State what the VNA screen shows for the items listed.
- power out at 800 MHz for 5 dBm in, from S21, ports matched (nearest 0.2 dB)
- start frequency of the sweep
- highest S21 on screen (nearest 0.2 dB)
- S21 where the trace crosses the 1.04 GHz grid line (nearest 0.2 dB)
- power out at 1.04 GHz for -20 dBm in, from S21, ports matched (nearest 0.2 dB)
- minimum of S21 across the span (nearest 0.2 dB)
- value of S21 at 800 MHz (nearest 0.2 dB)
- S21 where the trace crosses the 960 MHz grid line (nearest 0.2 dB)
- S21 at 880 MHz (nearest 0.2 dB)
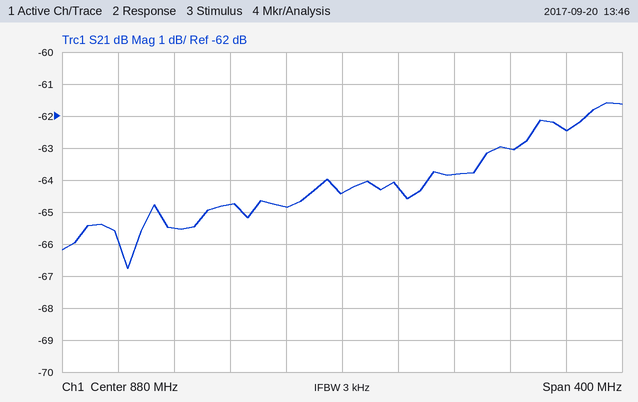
-59.8 dBm
680 MHz
-61.6 dB
-62.4 dB
-82.4 dBm
-66.8 dB
-64.8 dB
-63.8 dB
-64.4 dB
